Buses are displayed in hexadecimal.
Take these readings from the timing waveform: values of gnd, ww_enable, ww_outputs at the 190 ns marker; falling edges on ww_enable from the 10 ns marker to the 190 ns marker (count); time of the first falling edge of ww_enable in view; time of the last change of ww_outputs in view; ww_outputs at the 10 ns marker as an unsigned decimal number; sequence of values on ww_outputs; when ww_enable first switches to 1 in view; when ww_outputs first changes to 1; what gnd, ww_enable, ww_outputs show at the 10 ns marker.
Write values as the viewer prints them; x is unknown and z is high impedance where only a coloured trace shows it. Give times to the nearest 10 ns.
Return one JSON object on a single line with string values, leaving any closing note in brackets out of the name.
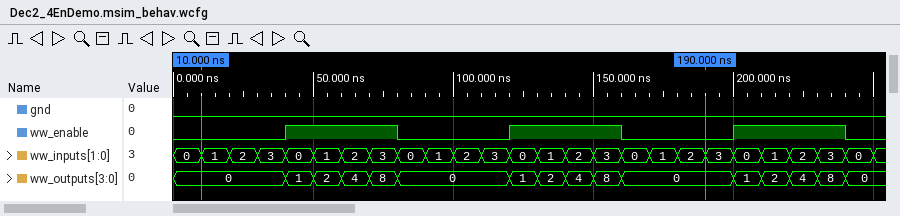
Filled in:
{"values of gnd, ww_enable, ww_outputs at the 190 ns marker": "gnd=0, ww_enable=0, ww_outputs=0", "falling edges on ww_enable from the 10 ns marker to the 190 ns marker": "2", "time of the first falling edge of ww_enable in view": "80 ns", "time of the last change of ww_outputs in view": "240 ns", "ww_outputs at the 10 ns marker as an unsigned decimal number": "0", "sequence of values on ww_outputs": "0, 1, 2, 4, 8, 0, 1, 2, 4, 8, 0, 1, 2, 4, 8, 0", "when ww_enable first switches to 1 in view": "40 ns", "when ww_outputs first changes to 1": "40 ns", "what gnd, ww_enable, ww_outputs show at the 10 ns marker": "gnd=0, ww_enable=0, ww_outputs=0"}
